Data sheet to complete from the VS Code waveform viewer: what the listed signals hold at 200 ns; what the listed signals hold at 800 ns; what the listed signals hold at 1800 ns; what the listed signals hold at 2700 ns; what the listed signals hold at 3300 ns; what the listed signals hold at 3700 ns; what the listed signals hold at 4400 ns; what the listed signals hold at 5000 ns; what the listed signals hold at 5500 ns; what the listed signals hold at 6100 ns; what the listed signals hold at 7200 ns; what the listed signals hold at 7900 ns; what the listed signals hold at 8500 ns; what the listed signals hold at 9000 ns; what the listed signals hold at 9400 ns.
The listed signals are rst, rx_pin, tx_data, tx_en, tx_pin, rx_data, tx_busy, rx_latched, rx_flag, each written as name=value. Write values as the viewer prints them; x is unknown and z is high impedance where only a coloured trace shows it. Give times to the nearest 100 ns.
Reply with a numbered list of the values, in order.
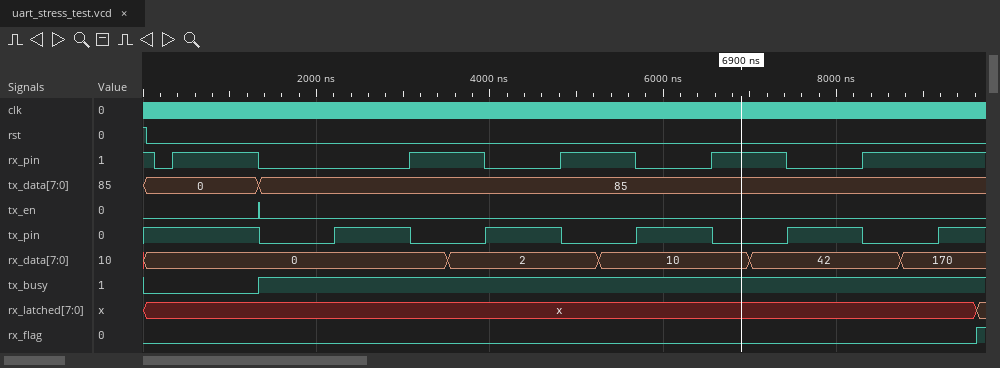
1. rst=0, rx_pin=0, tx_data=0, tx_en=0, tx_pin=1, rx_data=0, tx_busy=0, rx_latched=x, rx_flag=0
2. rst=0, rx_pin=1, tx_data=0, tx_en=0, tx_pin=1, rx_data=0, tx_busy=0, rx_latched=x, rx_flag=0
3. rst=0, rx_pin=0, tx_data=85, tx_en=0, tx_pin=0, rx_data=0, tx_busy=1, rx_latched=x, rx_flag=0
4. rst=0, rx_pin=0, tx_data=85, tx_en=0, tx_pin=1, rx_data=0, tx_busy=1, rx_latched=x, rx_flag=0
5. rst=0, rx_pin=1, tx_data=85, tx_en=0, tx_pin=0, rx_data=0, tx_busy=1, rx_latched=x, rx_flag=0
6. rst=0, rx_pin=1, tx_data=85, tx_en=0, tx_pin=0, rx_data=2, tx_busy=1, rx_latched=x, rx_flag=0
7. rst=0, rx_pin=0, tx_data=85, tx_en=0, tx_pin=1, rx_data=2, tx_busy=1, rx_latched=x, rx_flag=0
8. rst=0, rx_pin=1, tx_data=85, tx_en=0, tx_pin=0, rx_data=2, tx_busy=1, rx_latched=x, rx_flag=0
9. rst=0, rx_pin=1, tx_data=85, tx_en=0, tx_pin=0, rx_data=10, tx_busy=1, rx_latched=x, rx_flag=0
10. rst=0, rx_pin=0, tx_data=85, tx_en=0, tx_pin=1, rx_data=10, tx_busy=1, rx_latched=x, rx_flag=0
11. rst=0, rx_pin=1, tx_data=85, tx_en=0, tx_pin=0, rx_data=42, tx_busy=1, rx_latched=x, rx_flag=0
12. rst=0, rx_pin=0, tx_data=85, tx_en=0, tx_pin=1, rx_data=42, tx_busy=1, rx_latched=x, rx_flag=0
13. rst=0, rx_pin=1, tx_data=85, tx_en=0, tx_pin=0, rx_data=42, tx_busy=1, rx_latched=x, rx_flag=0
14. rst=0, rx_pin=1, tx_data=85, tx_en=0, tx_pin=0, rx_data=170, tx_busy=1, rx_latched=x, rx_flag=0
15. rst=0, rx_pin=1, tx_data=85, tx_en=0, tx_pin=1, rx_data=170, tx_busy=1, rx_latched=x, rx_flag=0
